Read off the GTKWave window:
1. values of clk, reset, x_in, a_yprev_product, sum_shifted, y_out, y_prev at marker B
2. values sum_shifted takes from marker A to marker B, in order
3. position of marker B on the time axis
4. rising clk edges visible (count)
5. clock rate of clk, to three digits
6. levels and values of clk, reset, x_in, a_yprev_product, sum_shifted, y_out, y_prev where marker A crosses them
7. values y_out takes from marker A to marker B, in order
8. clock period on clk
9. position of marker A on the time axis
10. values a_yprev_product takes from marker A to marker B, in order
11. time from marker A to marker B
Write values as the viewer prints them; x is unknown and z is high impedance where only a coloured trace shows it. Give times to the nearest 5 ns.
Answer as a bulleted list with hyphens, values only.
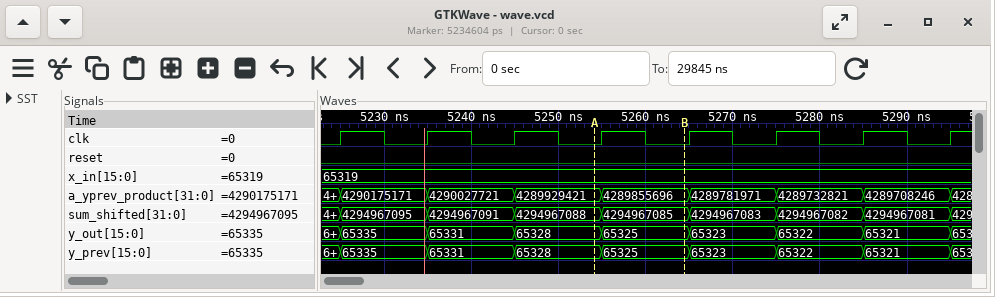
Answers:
- clk=0, reset=0, x_in=65319, a_yprev_product=4289855696, sum_shifted=4294967085, y_out=65325, y_prev=65325
- 4294967088, 4294967085
- 5265 ns
- 8
- 100 MHz
- clk=0, reset=0, x_in=65319, a_yprev_product=4289929421, sum_shifted=4294967088, y_out=65328, y_prev=65328
- 65328, 65325
- 10 ns
- 5255 ns
- 4289929421, 4289855696
- 10 ns
